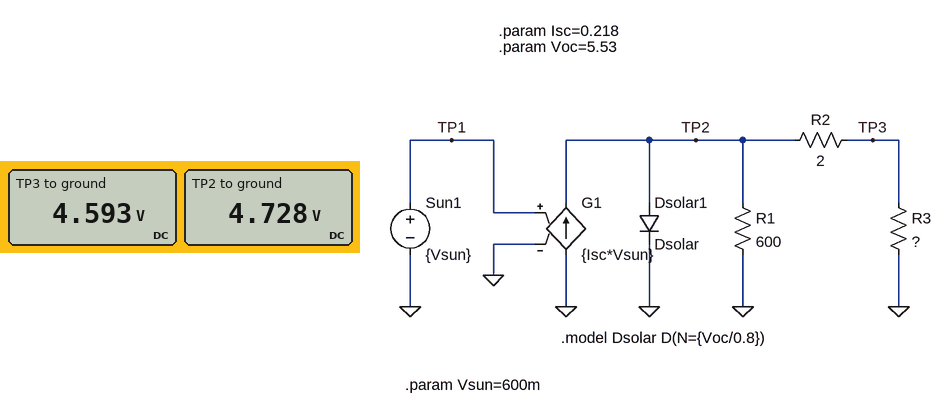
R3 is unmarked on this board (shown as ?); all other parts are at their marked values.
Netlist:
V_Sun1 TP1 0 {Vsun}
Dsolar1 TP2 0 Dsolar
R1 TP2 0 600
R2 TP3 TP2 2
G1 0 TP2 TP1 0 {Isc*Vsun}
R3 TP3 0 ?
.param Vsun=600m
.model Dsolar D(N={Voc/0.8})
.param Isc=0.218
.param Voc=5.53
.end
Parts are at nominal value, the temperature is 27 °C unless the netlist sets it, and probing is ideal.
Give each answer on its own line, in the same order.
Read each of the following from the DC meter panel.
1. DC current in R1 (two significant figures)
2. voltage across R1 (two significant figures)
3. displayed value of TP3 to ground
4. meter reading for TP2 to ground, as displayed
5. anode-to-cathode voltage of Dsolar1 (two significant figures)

7.9 mA
4.7 V
4.593 V
4.728 V
4.7 V
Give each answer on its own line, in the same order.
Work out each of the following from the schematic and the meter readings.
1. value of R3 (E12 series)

68 Ω
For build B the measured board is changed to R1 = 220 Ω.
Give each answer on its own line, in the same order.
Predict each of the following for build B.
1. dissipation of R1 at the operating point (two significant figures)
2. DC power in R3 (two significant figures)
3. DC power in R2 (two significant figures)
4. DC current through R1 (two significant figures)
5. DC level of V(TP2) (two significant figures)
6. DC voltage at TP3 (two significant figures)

79 mW
240 mW
7.1 mW
19 mA
4.2 V
4.0 V
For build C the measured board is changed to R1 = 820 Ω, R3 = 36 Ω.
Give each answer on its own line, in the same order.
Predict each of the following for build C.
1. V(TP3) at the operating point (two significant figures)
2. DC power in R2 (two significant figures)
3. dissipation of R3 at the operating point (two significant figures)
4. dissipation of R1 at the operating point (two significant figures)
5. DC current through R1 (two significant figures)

2.7 V
11 mW
200 mW
9.9 mW
3.5 mA
